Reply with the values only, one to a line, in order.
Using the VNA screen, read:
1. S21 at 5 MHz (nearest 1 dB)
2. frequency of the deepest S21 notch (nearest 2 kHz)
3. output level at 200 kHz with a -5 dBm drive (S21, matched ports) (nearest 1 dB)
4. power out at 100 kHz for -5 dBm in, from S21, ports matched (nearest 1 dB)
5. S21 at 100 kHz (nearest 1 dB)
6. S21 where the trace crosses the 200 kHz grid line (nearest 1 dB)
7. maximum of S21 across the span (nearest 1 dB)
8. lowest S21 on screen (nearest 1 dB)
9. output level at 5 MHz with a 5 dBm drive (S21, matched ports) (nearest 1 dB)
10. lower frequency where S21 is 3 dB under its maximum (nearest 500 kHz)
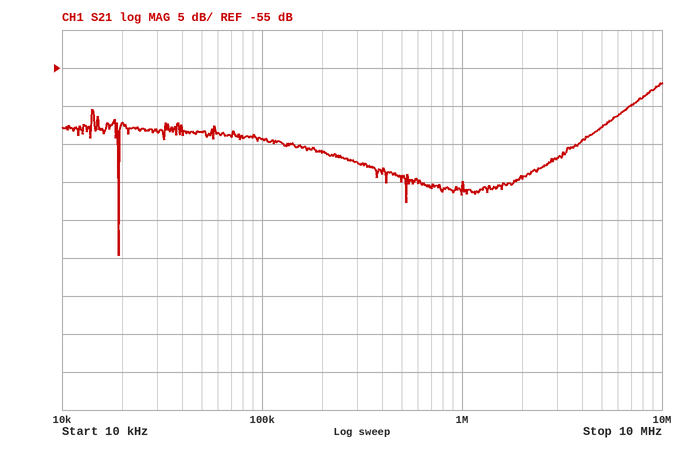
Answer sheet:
-63 dB
20 kHz
-71 dBm
-69 dBm
-64 dB
-66 dB
-57 dB
-80 dB
-58 dBm
7.0 MHz
